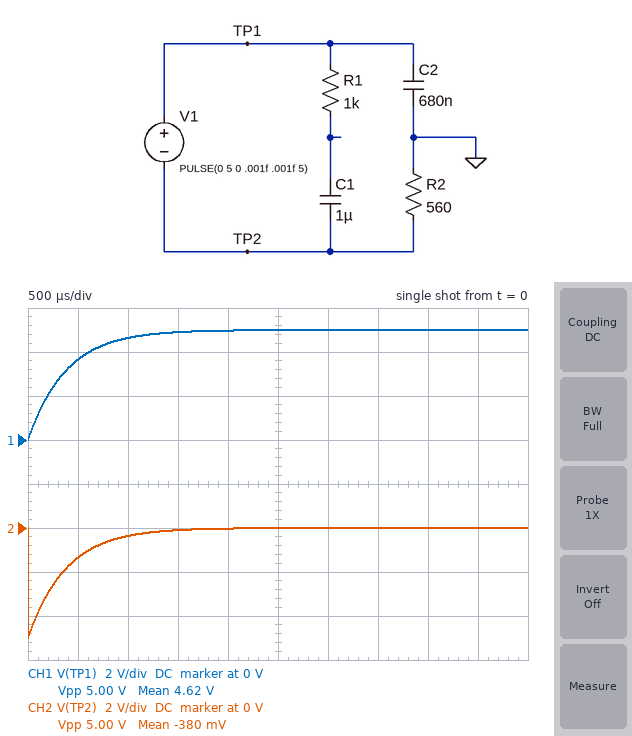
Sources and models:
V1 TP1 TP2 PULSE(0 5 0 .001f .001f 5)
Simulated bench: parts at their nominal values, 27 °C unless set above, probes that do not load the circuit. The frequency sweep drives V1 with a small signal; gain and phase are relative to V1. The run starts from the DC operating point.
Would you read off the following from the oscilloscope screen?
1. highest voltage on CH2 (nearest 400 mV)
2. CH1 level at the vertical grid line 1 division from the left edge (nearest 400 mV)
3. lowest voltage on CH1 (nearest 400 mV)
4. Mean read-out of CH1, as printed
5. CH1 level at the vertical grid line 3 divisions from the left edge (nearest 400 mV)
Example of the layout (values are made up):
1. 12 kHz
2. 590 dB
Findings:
1. 0 V
2. 3.6 V
3. 0 V
4. 4.62 V
5. 4.8 V
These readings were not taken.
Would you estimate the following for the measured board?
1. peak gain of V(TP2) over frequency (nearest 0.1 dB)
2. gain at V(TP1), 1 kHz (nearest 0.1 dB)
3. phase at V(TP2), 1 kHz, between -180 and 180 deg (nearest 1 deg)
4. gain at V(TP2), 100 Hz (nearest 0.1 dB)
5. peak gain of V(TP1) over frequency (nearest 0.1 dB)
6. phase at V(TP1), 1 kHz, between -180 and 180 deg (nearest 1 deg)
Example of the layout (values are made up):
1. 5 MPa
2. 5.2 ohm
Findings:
1. 0 dB
2. -8.3 dB
3. -157 deg
4. -12.7 dB
5. 0 dB
6. -67 deg
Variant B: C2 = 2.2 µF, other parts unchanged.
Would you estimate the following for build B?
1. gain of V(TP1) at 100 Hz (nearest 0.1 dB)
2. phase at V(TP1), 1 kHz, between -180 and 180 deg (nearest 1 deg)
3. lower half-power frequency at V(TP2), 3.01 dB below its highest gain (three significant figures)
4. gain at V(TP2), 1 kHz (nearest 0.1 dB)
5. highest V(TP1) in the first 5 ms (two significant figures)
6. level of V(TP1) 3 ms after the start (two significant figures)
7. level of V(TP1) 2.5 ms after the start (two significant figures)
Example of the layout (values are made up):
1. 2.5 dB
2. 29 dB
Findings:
1. -2.0 dB
2. -83 deg
3. 129 Hz
4. -0.1 dB
5. 4.9 V
6. 4.6 V
7. 4.3 V
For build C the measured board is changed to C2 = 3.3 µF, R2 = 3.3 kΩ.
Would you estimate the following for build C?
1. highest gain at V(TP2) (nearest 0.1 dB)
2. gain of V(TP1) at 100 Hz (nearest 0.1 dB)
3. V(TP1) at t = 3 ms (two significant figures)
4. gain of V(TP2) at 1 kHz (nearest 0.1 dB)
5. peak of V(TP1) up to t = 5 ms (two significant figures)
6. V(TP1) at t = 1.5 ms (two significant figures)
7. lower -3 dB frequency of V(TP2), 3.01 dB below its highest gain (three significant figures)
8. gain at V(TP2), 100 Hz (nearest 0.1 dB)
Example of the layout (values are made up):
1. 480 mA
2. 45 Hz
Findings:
1. 0 dB
2. -16.8 dB
3. 1.2 V
4. 0 dB
5. 1.8 V
6. 640 mV
7. 14.6 Hz
8. -0.1 dB
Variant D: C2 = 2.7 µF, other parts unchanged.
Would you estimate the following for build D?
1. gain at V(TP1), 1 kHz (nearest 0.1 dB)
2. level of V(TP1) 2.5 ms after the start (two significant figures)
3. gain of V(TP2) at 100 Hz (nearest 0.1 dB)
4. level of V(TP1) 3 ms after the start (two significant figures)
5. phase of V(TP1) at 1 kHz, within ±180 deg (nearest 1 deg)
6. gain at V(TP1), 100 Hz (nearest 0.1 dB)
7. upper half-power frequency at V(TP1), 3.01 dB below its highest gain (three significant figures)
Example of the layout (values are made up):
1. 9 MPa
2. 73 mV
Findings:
1. -19.6 dB
2. 4.0 V
3. -3.2 dB
4. 4.3 V
5. -84 deg
6. -2.8 dB
7. 105 Hz
